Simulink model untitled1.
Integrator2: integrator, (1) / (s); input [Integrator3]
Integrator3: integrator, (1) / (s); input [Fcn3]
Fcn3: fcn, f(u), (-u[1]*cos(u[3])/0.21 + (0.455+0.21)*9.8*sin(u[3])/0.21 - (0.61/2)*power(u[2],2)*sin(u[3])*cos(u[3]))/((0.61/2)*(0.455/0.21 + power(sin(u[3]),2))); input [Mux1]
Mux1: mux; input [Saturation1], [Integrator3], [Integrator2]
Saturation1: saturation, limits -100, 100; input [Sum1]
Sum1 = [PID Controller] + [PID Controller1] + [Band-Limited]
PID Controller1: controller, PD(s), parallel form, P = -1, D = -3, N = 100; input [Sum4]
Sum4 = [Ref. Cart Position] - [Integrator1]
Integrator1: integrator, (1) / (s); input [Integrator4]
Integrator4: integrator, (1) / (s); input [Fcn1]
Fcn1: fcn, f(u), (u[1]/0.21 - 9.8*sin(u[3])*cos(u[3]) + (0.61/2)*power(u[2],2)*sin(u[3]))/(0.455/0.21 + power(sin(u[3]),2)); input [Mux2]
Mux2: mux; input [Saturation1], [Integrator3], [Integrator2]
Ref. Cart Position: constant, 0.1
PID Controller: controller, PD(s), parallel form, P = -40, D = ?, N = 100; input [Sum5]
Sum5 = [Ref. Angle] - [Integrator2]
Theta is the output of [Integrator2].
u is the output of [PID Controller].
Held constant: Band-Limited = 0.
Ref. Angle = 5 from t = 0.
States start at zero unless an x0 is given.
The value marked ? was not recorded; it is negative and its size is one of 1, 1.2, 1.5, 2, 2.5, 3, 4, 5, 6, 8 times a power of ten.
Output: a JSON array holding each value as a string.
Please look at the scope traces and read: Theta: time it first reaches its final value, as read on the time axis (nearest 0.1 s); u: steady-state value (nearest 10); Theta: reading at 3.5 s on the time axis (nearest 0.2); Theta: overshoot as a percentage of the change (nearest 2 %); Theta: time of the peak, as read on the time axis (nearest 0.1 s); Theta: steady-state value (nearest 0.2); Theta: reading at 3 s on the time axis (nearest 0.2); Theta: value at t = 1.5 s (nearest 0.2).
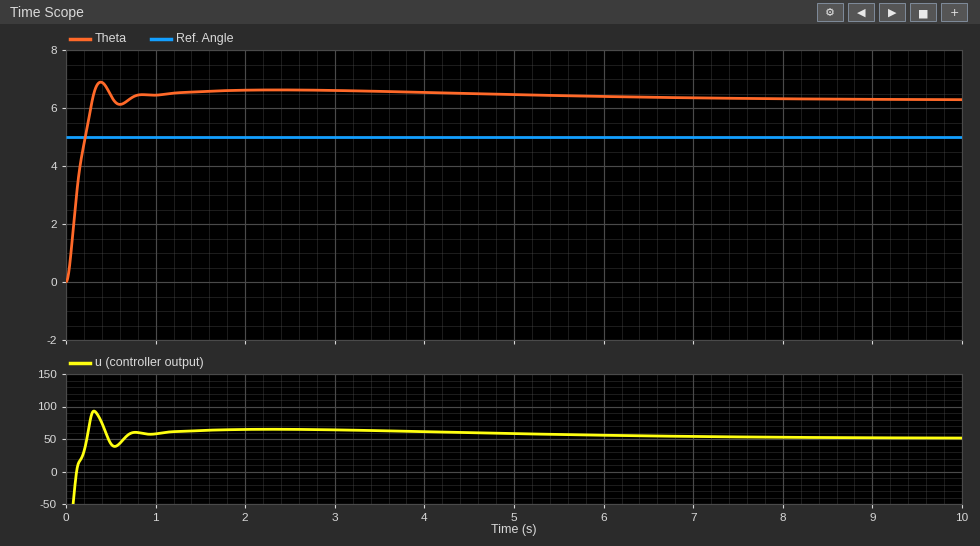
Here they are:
["0.3 s", "50", "6.6", "10 %", "0.4 s", "6.2", "6.6", "6.6"]
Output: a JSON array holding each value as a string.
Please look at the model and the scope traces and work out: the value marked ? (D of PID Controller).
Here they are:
["-2.5"]
